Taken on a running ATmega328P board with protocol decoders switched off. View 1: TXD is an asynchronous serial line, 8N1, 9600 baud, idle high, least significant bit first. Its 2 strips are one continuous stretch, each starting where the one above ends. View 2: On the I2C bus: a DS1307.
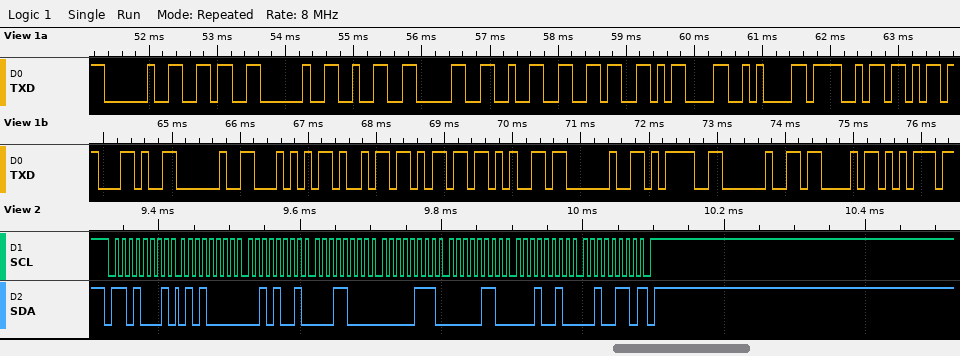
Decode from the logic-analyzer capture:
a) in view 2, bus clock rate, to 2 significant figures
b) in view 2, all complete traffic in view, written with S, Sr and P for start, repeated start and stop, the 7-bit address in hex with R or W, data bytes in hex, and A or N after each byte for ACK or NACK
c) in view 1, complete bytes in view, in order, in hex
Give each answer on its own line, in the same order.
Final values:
100 kHz
S 68R A 50 A 29 A 18 A 07 A 06 A 12 A 26 N P
0x20 0x36 0x20 0x32 0x30 0x32 0x36 0x0D 0x0A 0x4F 0x6B 0x2C 0x20 0x54 0x69 0x6D 0x65 0x20 0x3D 0x20 0x43 0x75
